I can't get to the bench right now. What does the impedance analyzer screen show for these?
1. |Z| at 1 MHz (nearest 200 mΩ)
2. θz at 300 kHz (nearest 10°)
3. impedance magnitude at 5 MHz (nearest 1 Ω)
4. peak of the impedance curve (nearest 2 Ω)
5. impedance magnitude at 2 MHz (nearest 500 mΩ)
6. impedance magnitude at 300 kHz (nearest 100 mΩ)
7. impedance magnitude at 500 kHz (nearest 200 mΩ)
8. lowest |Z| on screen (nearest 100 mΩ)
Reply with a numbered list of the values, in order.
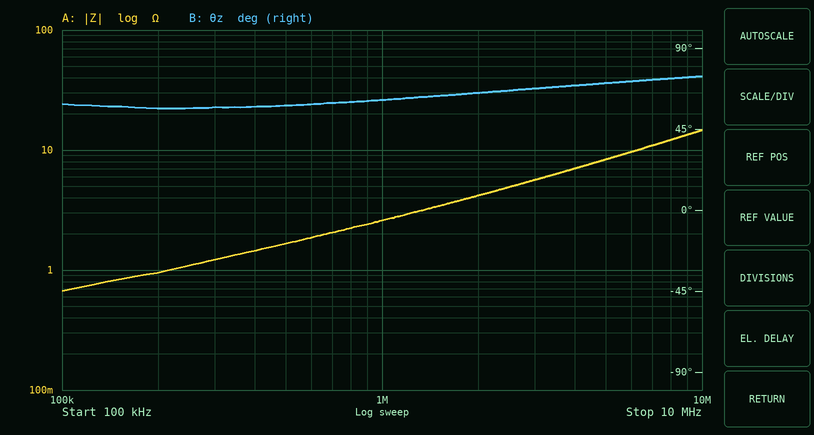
1. 2.6 Ω
2. 60°
3. 8 Ω
4. 14 Ω
5. 4.0 Ω
6. 1.2 Ω
7. 1.6 Ω
8. 700 mΩ
